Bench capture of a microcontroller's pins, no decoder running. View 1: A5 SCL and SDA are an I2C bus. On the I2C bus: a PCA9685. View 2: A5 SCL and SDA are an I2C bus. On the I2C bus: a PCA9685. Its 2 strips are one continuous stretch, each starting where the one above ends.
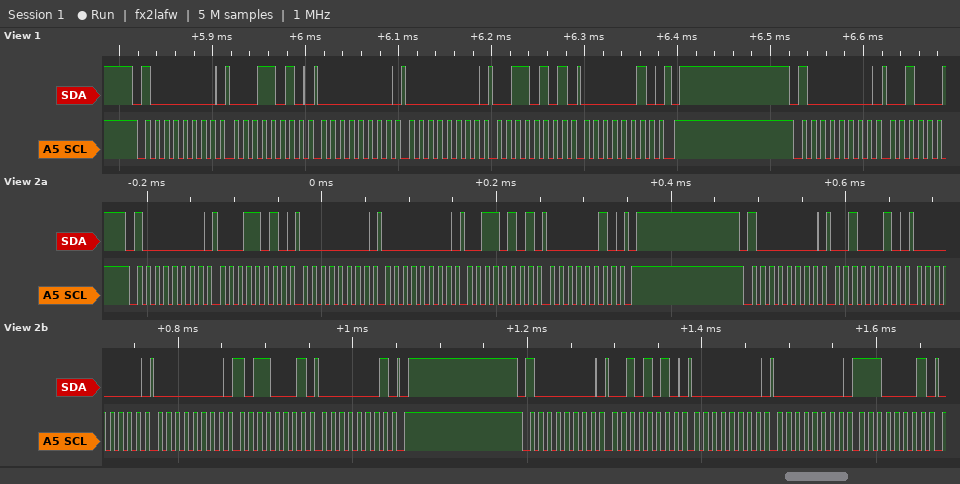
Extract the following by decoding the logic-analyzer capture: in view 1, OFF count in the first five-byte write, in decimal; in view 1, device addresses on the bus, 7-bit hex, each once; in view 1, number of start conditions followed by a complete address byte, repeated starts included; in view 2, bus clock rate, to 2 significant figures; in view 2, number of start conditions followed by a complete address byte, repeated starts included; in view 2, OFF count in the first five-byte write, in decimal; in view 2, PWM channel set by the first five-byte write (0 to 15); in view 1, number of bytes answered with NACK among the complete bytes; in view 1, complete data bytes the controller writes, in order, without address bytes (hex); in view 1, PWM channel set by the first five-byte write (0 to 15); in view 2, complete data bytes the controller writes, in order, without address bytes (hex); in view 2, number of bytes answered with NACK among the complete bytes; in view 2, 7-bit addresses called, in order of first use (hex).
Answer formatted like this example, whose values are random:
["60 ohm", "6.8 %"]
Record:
["565", "0x40", "2", "100 kHz", "3", "565", "5", "0", "1A 00 00 35 02", "5", "1A 00 00 35 02 22 00 00 B1 01 2A 00 00 E1", "0", "0x40"]
